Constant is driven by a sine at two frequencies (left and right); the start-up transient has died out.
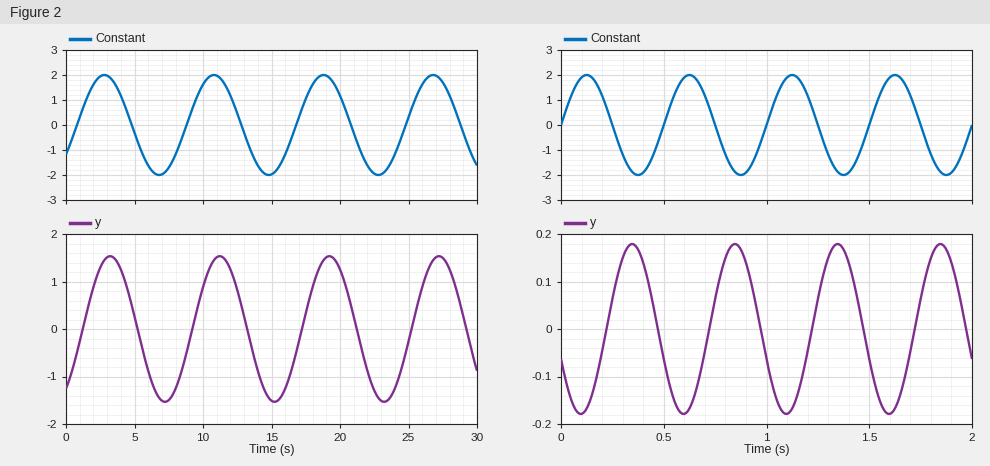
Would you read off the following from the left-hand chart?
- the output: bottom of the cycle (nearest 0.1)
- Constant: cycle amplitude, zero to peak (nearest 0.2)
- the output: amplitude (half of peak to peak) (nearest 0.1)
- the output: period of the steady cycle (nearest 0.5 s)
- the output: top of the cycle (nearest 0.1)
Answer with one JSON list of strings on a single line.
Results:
["-1.5", "2.0", "1.5", "8.0 s", "1.5"]
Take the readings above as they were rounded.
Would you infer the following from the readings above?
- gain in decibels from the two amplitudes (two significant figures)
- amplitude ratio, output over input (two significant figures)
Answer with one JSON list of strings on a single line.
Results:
["-2.5 dB", "0.75"]
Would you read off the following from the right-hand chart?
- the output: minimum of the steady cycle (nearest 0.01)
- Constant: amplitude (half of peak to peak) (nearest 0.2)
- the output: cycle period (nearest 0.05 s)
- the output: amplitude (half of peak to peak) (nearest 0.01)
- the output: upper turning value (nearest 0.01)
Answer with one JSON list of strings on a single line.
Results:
["-0.18", "2.0", "0.50 s", "0.18", "0.18"]
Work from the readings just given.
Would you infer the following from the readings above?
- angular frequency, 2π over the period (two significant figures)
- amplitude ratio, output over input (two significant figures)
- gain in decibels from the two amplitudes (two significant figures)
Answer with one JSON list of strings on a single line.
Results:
["13 rad/s", "0.090", "-21 dB"]
